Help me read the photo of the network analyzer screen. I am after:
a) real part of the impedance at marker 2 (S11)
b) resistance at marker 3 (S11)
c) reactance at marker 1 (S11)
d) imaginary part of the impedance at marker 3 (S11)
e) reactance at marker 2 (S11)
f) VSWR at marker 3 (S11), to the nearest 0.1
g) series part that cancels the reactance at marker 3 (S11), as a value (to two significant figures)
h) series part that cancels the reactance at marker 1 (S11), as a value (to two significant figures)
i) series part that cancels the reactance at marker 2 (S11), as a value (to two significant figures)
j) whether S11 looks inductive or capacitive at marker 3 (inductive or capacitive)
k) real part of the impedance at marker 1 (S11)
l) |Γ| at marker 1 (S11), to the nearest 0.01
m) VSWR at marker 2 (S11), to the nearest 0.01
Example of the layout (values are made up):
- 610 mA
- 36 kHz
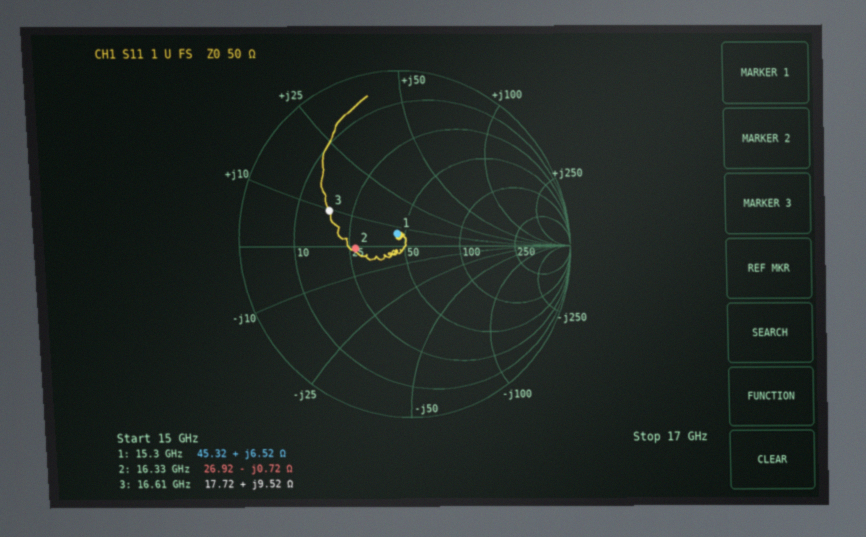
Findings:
- 26.92 Ω
- 17.72 Ω
- +6.52 Ω
- +9.52 Ω
- -0.72 Ω
- 2.9
- 1.0 pF
- 1.6 pF
- 7.0 pH
- inductive
- 45.32 Ω
- 0.08
- 1.86
